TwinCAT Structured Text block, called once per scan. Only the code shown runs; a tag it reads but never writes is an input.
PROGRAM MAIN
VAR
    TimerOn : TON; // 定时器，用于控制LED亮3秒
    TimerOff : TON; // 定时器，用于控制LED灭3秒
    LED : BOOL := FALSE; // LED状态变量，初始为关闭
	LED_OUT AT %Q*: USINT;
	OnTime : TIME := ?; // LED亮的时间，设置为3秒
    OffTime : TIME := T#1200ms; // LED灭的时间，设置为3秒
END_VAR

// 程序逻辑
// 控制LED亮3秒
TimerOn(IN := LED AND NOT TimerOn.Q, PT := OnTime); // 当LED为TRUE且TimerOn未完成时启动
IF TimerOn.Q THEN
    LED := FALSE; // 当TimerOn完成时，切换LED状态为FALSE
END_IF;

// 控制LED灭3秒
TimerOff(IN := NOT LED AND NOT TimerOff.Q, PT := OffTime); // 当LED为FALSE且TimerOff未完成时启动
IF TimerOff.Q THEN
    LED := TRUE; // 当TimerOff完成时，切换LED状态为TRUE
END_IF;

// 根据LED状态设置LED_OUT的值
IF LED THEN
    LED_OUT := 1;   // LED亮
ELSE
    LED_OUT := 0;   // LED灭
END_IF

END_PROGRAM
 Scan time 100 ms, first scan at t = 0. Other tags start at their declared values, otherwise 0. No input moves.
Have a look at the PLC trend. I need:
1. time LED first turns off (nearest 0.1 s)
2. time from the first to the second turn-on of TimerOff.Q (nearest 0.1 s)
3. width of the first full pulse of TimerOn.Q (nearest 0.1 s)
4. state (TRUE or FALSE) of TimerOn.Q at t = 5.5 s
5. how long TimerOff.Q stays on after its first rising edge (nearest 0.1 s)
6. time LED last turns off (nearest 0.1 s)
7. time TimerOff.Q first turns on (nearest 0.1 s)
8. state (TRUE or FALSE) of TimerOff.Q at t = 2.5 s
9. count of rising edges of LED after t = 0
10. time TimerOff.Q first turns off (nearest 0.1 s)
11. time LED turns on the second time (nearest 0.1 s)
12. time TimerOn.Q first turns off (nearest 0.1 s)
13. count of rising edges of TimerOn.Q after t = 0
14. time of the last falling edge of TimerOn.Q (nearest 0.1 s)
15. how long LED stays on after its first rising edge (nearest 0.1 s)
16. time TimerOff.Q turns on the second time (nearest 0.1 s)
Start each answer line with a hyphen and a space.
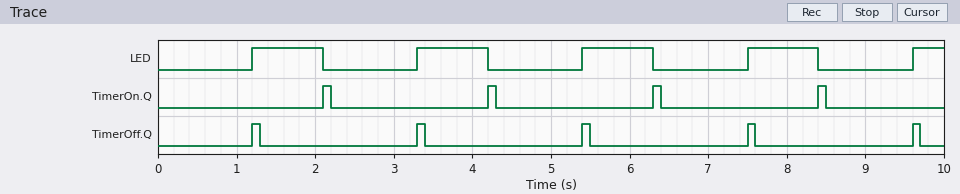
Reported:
- 2.1 s
- 2.1 s
- 0.1 s
- FALSE
- 0.1 s
- 8.4 s
- 1.2 s
- FALSE
- 5
- 1.3 s
- 3.3 s
- 2.2 s
- 4
- 8.5 s
- 0.9 s
- 3.3 s
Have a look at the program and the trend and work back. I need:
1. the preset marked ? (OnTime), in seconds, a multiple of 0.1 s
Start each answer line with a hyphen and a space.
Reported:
- 0.8 s
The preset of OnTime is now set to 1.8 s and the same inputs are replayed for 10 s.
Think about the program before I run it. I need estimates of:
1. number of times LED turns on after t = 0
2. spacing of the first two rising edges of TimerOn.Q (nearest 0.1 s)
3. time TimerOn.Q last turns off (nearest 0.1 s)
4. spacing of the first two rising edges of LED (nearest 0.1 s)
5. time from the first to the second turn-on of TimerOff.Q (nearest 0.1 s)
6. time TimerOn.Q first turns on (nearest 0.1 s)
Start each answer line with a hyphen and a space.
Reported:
- 3
- 3.1 s
- 9.4 s
- 3.1 s
- 3.1 s
- 3.1 s
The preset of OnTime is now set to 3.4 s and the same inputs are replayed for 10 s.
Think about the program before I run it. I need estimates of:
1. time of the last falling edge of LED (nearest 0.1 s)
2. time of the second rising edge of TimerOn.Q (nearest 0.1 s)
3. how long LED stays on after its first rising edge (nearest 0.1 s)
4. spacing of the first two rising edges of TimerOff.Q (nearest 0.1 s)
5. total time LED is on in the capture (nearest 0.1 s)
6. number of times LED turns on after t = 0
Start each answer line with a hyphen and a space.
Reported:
- 9.4 s
- 9.4 s
- 3.5 s
- 4.7 s
- 7.0 s
- 2
